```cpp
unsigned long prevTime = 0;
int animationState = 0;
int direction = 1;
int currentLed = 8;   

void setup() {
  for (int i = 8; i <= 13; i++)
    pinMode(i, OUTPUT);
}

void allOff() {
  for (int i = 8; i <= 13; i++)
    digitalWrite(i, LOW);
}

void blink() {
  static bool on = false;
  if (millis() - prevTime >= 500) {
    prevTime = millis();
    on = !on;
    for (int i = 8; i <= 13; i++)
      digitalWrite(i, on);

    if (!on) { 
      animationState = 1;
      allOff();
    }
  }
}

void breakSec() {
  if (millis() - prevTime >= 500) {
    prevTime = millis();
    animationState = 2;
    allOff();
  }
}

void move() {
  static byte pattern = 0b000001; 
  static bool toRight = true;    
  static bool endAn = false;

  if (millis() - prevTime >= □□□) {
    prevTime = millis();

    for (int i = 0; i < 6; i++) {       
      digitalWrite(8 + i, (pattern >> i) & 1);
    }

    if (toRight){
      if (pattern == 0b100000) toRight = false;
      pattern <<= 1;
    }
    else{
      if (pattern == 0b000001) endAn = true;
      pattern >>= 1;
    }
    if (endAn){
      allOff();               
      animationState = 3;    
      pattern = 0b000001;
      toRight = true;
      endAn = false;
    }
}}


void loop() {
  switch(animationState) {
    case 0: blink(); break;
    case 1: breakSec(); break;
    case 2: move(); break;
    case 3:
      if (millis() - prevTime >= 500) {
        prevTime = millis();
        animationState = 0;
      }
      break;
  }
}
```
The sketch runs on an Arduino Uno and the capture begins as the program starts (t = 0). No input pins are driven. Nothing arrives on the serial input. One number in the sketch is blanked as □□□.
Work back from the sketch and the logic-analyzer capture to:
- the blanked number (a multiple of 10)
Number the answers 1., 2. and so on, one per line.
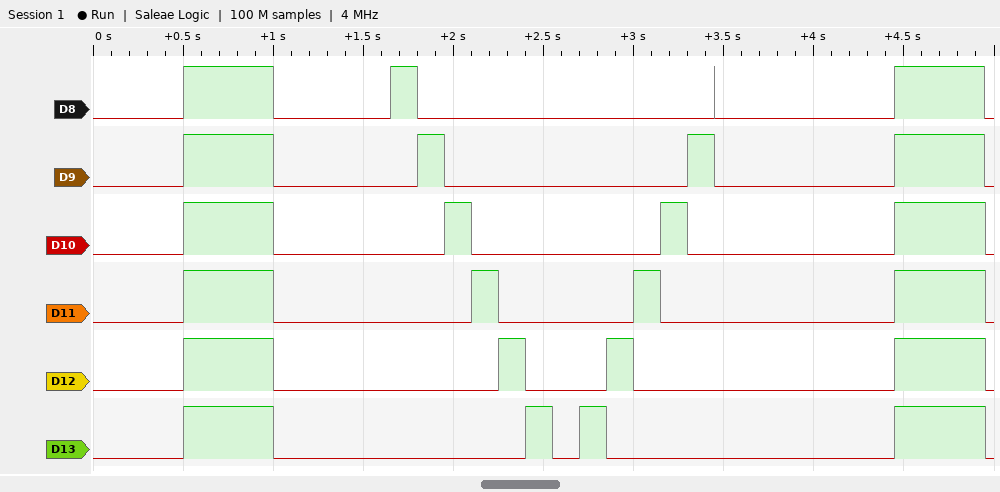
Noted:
1. 150
